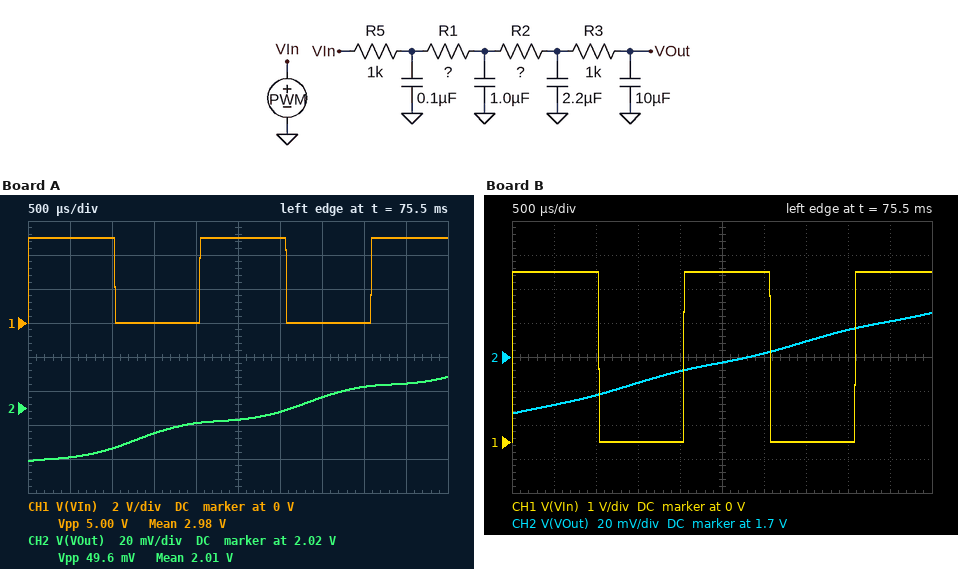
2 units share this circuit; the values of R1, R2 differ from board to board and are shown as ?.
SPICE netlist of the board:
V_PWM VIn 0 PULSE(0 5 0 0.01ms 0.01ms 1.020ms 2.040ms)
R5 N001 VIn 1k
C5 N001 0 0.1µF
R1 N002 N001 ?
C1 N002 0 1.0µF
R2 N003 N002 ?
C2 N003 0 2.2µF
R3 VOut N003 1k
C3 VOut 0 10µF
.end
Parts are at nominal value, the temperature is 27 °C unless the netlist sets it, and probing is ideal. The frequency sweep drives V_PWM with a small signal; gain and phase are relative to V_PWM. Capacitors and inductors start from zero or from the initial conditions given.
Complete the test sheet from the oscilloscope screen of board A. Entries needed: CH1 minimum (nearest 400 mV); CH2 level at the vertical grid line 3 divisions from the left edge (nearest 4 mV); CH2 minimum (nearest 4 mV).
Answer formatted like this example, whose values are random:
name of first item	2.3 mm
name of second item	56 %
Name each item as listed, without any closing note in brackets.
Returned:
CH1 minimum	0 V
CH2 level at the vertical grid line 3 divisions from the left edge	2.004 V
CH2 minimum	1.988 V
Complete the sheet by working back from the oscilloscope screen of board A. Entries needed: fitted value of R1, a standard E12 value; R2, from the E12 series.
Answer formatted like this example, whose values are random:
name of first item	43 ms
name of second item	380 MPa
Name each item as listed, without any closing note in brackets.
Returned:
fitted value of R1, a standard E12 value	1.5 kΩ
R2, from the E12 series	560 Ω
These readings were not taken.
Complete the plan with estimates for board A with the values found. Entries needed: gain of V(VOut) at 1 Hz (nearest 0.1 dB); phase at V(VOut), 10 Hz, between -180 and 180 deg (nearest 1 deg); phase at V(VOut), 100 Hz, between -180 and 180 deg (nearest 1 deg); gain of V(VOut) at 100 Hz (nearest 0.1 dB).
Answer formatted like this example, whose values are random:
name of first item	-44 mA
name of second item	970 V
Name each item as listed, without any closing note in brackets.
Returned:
gain of V(VOut) at 1 Hz	-0.4 dB
phase at V(VOut), 10 Hz, between -180 and 180 deg	-80 deg
phase at V(VOut), 100 Hz, between -180 and 180 deg	-153 deg
gain of V(VOut) at 100 Hz	-33.7 dB
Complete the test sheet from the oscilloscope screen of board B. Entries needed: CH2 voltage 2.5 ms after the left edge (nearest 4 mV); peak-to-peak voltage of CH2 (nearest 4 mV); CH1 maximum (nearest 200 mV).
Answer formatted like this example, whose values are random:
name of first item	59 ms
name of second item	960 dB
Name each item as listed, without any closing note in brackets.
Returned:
CH2 voltage 2.5 ms after the left edge	1.696 V
peak-to-peak voltage of CH2	60 mV
CH1 maximum	5.0 V
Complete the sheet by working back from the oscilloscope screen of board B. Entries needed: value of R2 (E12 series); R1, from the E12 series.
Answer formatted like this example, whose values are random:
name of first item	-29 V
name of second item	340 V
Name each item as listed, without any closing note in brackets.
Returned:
value of R2	1.5 kΩ
R1, from the E12 series	2.2 kΩ
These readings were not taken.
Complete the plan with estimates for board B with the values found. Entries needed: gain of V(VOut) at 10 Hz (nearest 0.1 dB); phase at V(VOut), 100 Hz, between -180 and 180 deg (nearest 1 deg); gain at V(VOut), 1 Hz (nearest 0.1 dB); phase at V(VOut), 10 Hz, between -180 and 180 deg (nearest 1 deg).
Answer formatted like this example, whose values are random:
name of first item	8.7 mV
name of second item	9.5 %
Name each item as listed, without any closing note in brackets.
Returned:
gain of V(VOut) at 10 Hz	-12.9 dB
phase at V(VOut), 100 Hz, between -180 and 180 deg	-169 deg
gain at V(VOut), 1 Hz	-0.7 dB
phase at V(VOut), 10 Hz, between -180 and 180 deg	-87 deg
